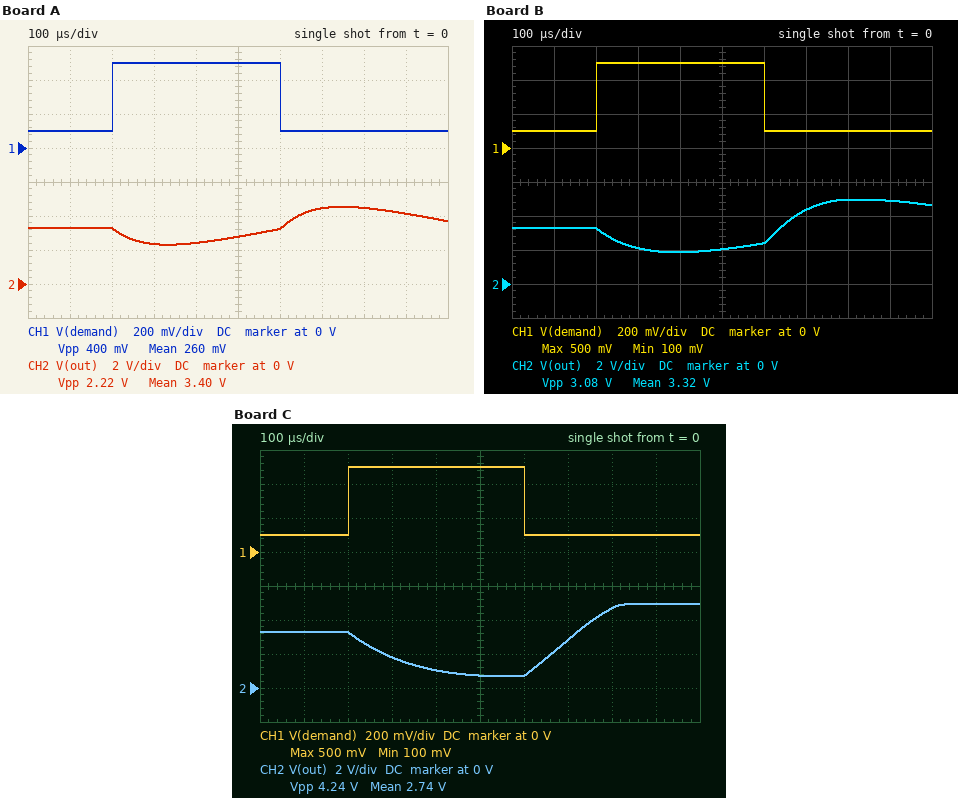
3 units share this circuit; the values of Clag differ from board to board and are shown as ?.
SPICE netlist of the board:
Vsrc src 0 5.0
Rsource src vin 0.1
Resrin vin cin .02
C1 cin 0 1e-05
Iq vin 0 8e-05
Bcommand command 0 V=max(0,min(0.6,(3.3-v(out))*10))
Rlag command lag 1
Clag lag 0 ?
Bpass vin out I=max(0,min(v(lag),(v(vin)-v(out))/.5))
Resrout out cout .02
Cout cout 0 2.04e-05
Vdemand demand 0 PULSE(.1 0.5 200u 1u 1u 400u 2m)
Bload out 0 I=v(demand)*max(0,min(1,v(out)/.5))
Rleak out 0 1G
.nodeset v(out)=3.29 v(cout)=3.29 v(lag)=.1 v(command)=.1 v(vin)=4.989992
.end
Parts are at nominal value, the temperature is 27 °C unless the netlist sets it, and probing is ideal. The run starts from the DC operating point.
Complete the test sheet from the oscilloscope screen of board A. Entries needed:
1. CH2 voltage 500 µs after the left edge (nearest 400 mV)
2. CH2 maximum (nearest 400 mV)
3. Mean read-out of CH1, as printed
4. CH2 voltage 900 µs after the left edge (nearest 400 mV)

2.8 V
4.4 V
260 mV
4.0 V
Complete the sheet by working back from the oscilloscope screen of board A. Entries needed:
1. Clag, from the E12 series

82 µF
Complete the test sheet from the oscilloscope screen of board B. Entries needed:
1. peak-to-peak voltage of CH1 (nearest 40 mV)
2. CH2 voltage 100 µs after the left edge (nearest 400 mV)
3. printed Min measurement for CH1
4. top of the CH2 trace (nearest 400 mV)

400 mV
3.2 V
100 mV
4.8 V
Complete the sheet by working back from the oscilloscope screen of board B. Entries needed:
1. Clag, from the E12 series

120 µF
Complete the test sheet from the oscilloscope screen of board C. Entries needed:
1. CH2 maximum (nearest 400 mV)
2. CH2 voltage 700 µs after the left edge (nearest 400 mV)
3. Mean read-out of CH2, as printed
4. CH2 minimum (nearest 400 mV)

4.8 V
2.8 V
2.74 V
800 mV
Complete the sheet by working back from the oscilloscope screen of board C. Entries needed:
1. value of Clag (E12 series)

220 µF
